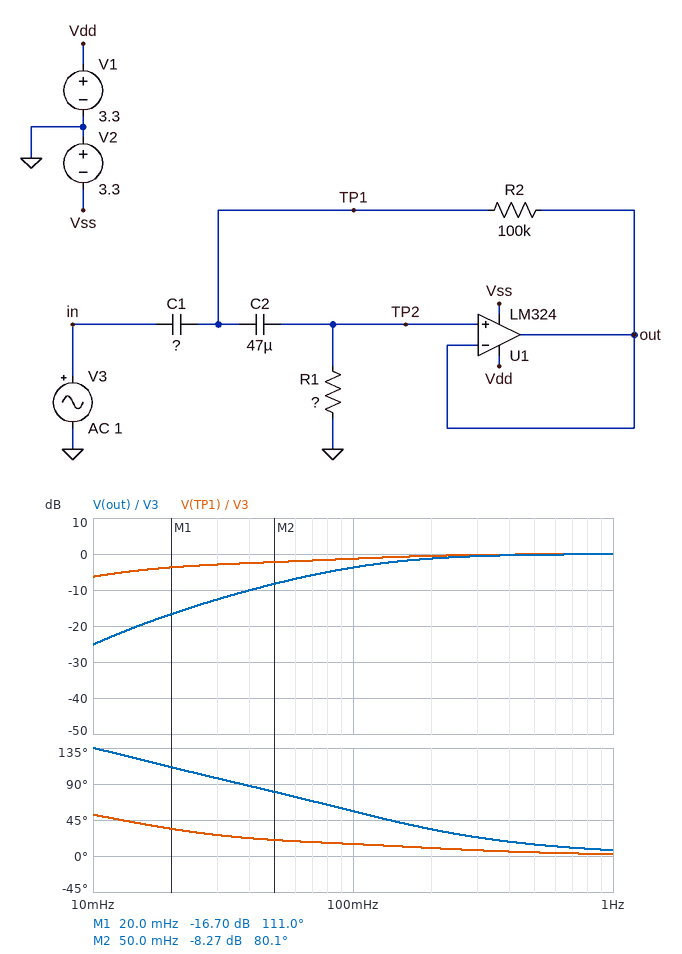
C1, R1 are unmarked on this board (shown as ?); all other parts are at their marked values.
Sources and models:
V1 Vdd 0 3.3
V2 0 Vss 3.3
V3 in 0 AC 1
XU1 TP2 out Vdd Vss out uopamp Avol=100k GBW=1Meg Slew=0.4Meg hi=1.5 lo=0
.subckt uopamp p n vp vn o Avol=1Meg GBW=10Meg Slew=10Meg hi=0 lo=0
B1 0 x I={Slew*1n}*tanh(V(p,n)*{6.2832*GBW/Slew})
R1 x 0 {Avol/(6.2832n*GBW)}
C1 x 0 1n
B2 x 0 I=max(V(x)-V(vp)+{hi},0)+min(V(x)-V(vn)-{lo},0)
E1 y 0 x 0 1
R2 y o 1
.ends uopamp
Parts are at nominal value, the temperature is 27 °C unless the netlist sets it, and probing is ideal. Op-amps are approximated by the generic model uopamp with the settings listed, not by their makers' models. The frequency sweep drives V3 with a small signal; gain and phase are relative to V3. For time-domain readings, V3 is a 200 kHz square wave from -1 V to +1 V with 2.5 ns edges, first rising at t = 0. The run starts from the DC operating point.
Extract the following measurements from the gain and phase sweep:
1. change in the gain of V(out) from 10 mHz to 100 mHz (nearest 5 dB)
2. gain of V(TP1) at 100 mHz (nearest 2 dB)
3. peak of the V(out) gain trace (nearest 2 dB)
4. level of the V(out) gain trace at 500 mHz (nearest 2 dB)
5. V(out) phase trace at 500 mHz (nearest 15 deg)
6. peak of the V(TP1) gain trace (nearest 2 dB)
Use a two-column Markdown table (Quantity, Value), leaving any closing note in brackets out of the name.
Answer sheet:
| Quantity | Value |
|---|---|
| change in the gain of V(out) from 10 mHz to 100 mHz | 20 dB |
| gain of V(TP1) at 100 mHz | -2 dB |
| peak of the V(out) gain trace | 0 dB |
| level of the V(out) gain trace at 500 mHz | 0 dB |
| V(out) phase trace at 500 mHz | 15 deg |
| peak of the V(TP1) gain trace | 0 dB |
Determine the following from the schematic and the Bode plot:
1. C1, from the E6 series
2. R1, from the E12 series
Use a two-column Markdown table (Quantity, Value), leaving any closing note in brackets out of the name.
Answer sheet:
| Quantity | Value |
|---|---|
| C1, from the E6 series | 100 µF |
| R1, from the E12 series | 39 kΩ |
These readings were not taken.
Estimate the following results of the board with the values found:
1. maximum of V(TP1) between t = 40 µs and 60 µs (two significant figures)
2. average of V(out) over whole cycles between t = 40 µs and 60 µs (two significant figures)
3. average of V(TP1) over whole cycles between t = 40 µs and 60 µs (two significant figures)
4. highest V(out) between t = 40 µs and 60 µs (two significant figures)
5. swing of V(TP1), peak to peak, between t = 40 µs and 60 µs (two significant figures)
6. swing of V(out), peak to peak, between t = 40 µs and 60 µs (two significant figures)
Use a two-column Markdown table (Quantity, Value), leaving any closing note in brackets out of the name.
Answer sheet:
| Quantity | Value |
|---|---|
| maximum of V(TP1) between t = 40 µs and 60 µs | 2.0 V |
| average of V(out) over whole cycles between t = 40 µs and 60 µs | 600 mV |
| average of V(TP1) over whole cycles between t = 40 µs and 60 µs | 1.0 V |
| highest V(out) between t = 40 µs and 60 µs | 1.1 V |
| swing of V(TP1), peak to peak, between t = 40 µs and 60 µs | 2.0 V |
| swing of V(out), peak to peak, between t = 40 µs and 60 µs | 1.0 V |
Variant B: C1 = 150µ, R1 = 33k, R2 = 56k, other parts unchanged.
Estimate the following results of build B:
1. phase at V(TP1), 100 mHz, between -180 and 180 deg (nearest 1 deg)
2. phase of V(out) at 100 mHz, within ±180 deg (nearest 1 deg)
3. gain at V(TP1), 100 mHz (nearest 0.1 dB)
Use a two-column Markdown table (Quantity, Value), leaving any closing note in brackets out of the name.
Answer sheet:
| Quantity | Value |
|---|---|
| phase at V(TP1), 100 mHz, between -180 and 180 deg | 13 deg |
| phase of V(out) at 100 mHz, within ±180 deg | 59 deg |
| gain at V(TP1), 100 mHz | -0.8 dB |
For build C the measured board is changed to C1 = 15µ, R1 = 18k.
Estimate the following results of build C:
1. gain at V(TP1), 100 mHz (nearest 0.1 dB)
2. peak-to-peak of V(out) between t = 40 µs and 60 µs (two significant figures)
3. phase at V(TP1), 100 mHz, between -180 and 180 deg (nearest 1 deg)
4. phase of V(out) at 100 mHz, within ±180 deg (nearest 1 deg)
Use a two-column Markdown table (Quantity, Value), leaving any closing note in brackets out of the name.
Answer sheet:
| Quantity | Value |
|---|---|
| gain at V(TP1), 100 mHz | -11.3 dB |
| peak-to-peak of V(out) between t = 40 µs and 60 µs | 1.0 V |
| phase at V(TP1), 100 mHz, between -180 and 180 deg | 35 deg |
| phase of V(out) at 100 mHz, within ±180 deg | 97 deg |
